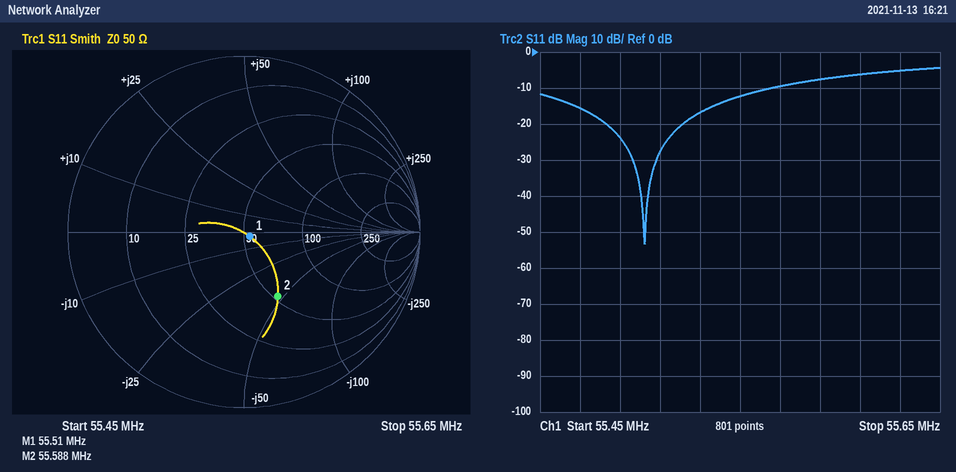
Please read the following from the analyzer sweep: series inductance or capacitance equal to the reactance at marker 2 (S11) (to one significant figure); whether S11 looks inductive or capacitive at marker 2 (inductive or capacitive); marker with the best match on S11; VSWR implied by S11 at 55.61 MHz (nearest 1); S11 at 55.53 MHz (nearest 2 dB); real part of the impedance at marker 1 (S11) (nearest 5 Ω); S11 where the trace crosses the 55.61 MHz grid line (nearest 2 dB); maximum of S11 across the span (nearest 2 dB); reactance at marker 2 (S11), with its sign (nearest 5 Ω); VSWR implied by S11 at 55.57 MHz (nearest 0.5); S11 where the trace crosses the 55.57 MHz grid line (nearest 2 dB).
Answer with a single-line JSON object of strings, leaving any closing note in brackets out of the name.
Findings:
{"series inductance or capacitance equal to the reactance at marker 2 (S11)": "60 pF", "whether S11 looks inductive or capacitive at marker 2": "capacitive", "marker with the best match on S11": "marker 1", "VSWR implied by S11 at 55.61 MHz": "3", "S11 at 55.53 MHz": "-16 dB", "real part of the impedance at marker 1 (S11)": "55 Ω", "S11 where the trace crosses the 55.61 MHz grid line": "-6 dB", "maximum of S11 across the span": "-4 dB", "reactance at marker 2 (S11), with its sign": "-45 Ω", "VSWR implied by S11 at 55.57 MHz": "2.0", "S11 where the trace crosses the 55.57 MHz grid line": "-10 dB"}
